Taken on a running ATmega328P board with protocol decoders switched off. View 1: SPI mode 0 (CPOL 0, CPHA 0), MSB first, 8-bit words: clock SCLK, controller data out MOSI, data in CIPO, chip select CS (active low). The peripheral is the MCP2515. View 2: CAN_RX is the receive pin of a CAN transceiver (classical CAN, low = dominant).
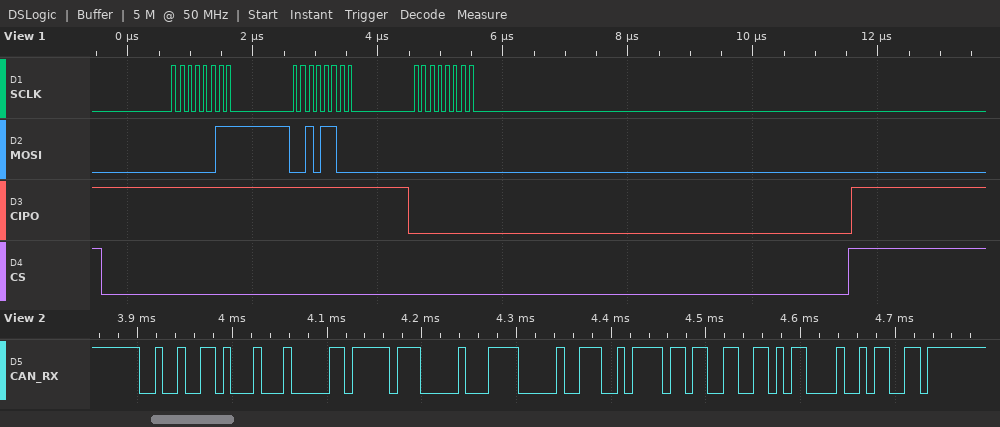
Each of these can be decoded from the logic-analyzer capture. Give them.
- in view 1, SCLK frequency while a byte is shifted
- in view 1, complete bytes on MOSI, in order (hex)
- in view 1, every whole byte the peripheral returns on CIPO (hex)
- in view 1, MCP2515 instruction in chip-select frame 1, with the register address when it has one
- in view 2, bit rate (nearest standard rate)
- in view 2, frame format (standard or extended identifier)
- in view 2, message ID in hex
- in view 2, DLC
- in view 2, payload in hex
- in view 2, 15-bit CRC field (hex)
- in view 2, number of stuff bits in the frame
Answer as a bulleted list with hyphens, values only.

- 8 MHz
- 03 2C 00
- FF FF 00
- READ 0x2C
- 125 kbit/s
- standard
- 0x24D
- 8
- 82 FF 00 F0 1C BD B3 35
- 0x4259
- 4
